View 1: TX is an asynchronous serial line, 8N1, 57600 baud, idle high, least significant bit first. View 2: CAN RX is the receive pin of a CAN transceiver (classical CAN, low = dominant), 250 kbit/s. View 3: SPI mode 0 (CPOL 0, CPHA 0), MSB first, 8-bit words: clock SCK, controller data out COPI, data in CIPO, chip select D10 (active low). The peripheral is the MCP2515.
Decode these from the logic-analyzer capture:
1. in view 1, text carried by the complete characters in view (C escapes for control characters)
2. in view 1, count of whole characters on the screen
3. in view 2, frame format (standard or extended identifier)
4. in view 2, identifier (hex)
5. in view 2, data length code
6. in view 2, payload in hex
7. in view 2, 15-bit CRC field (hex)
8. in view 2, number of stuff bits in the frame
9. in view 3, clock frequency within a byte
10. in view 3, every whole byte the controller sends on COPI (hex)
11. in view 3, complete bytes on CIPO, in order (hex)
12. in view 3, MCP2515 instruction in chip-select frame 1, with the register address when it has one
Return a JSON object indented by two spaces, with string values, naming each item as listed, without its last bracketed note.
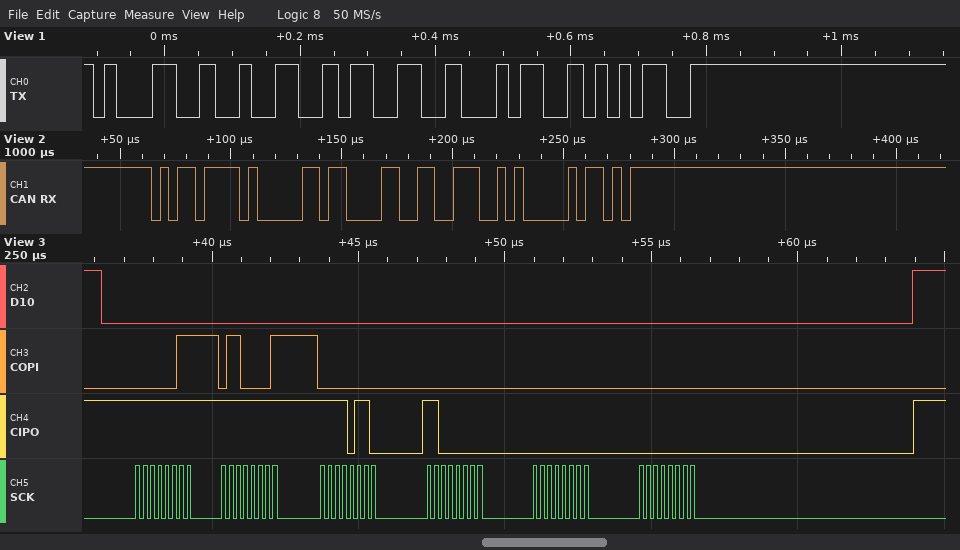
{
  "in view 1, text carried by the complete characters in view": "\"12345\"",
  "in view 1, count of whole characters on the screen": "5",
  "in view 2, frame format": "standard",
  "in view 2, identifier": "0x5BD",
  "in view 2, data length code": "2",
  "in view 2, payload in hex": "C3 33",
  "in view 2, 15-bit CRC field": "0x4A06",
  "in view 2, number of stuff bits in the frame": "2",
  "in view 3, clock frequency within a byte": "4 MHz",
  "in view 3, every whole byte the controller sends on COPI": "03 61 00 00 00 00",
  "in view 3, complete bytes on CIPO, in order": "FF FF F6 C0 00 00",
  "in view 3, MCP2515 instruction in chip-select frame 1, with the register address when it has one": "READ 0x61"
}
